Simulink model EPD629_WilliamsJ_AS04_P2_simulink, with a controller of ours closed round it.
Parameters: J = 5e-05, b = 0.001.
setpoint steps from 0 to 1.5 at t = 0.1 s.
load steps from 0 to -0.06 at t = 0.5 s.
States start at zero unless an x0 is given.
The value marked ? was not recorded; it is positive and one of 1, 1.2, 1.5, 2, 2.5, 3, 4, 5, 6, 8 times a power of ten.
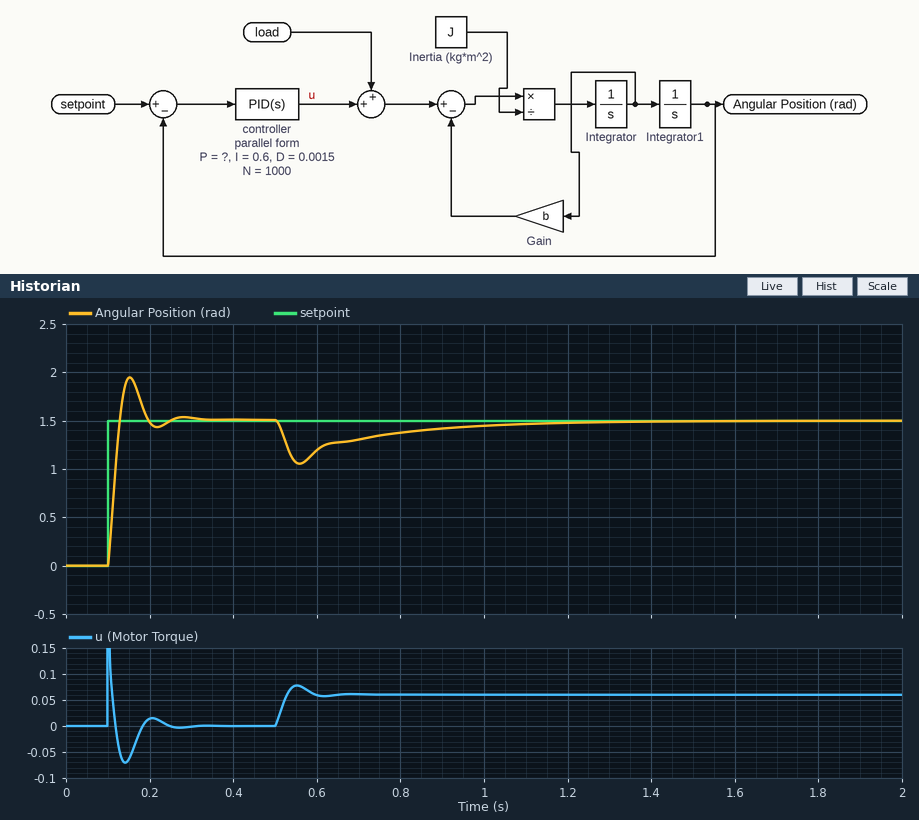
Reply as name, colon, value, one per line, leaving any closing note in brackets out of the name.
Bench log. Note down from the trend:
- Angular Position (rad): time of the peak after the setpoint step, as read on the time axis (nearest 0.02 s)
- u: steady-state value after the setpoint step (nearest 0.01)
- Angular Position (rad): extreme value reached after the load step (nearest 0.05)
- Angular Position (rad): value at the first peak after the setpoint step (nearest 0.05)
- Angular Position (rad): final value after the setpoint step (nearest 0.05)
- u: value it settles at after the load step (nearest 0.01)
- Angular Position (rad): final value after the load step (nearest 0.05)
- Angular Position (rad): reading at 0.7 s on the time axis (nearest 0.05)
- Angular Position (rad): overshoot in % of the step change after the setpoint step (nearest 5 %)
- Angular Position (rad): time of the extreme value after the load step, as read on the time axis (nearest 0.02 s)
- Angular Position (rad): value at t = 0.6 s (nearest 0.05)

Angular Position (rad): time of the peak after the setpoint step, as read on the time axis: 0.16 s
u: steady-state value after the setpoint step: 0.00
Angular Position (rad): extreme value reached after the load step: 1.05
Angular Position (rad): value at the first peak after the setpoint step: 1.95
Angular Position (rad): final value after the setpoint step: 1.50
u: value it settles at after the load step: 0.06
Angular Position (rad): final value after the load step: 1.50
Angular Position (rad): reading at 0.7 s on the time axis: 1.30
Angular Position (rad): overshoot in % of the step change after the setpoint step: 30 %
Angular Position (rad): time of the extreme value after the load step, as read on the time axis: 0.56 s
Angular Position (rad): value at t = 0.6 s: 1.20
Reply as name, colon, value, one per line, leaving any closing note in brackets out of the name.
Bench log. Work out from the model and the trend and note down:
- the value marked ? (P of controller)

the value marked ?: 0.15
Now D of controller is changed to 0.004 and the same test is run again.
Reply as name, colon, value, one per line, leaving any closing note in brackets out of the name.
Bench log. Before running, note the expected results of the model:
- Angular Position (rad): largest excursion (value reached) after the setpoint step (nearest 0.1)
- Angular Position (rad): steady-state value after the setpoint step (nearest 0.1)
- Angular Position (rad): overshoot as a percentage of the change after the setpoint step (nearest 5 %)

Angular Position (rad): largest excursion (value reached) after the setpoint step: 1.6
Angular Position (rad): steady-state value after the setpoint step: 1.5
Angular Position (rad): overshoot as a percentage of the change after the setpoint step: 10 %
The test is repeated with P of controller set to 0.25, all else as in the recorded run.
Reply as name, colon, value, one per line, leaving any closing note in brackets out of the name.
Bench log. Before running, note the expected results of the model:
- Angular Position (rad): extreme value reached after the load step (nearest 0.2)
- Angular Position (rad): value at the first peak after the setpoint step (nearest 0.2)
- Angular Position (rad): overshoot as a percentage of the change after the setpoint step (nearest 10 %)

Angular Position (rad): extreme value reached after the load step: 1.2
Angular Position (rad): value at the first peak after the setpoint step: 2.0
Angular Position (rad): overshoot as a percentage of the change after the setpoint step: 40 %
